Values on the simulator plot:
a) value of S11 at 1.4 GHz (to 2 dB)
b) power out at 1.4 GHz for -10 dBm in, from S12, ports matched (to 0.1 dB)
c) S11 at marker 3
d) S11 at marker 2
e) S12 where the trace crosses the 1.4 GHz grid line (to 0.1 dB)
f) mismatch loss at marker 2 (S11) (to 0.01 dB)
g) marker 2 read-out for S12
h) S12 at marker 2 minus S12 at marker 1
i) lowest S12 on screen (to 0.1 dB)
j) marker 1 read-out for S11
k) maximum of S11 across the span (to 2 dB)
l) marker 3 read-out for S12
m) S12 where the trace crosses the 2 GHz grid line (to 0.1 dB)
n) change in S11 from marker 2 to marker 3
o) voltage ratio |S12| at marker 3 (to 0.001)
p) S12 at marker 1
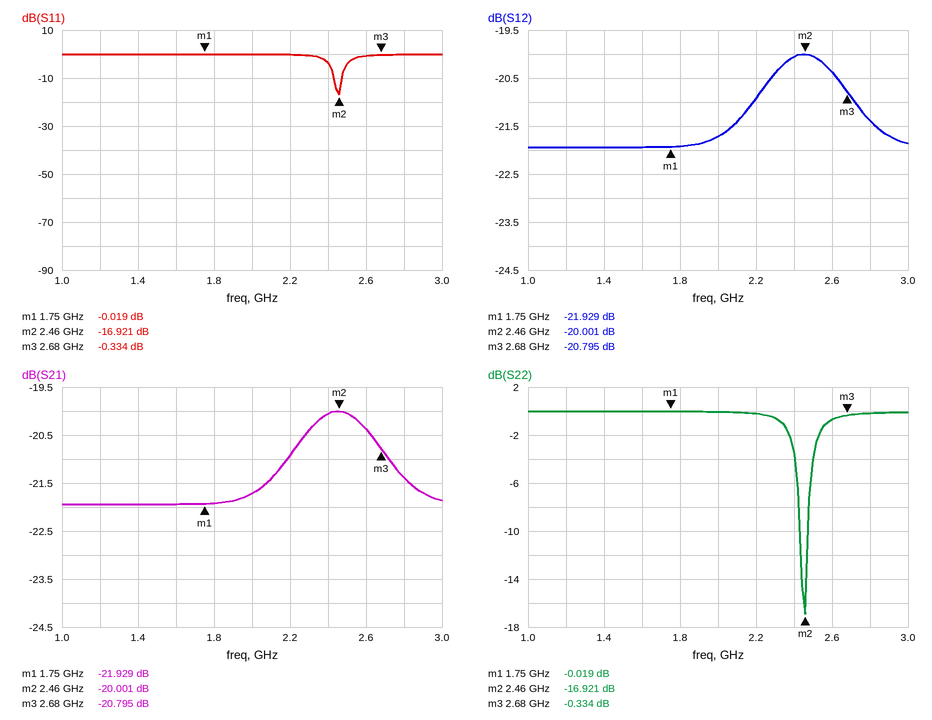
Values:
0 dB
-31.9 dBm
-0.334 dB
-16.921 dB
-21.9 dB
0.09 dB
-20.001 dB
1.928 dB
-21.9 dB
-0.019 dB
0 dB
-20.795 dB
-21.7 dB
16.587 dB
0.091
-21.929 dB
